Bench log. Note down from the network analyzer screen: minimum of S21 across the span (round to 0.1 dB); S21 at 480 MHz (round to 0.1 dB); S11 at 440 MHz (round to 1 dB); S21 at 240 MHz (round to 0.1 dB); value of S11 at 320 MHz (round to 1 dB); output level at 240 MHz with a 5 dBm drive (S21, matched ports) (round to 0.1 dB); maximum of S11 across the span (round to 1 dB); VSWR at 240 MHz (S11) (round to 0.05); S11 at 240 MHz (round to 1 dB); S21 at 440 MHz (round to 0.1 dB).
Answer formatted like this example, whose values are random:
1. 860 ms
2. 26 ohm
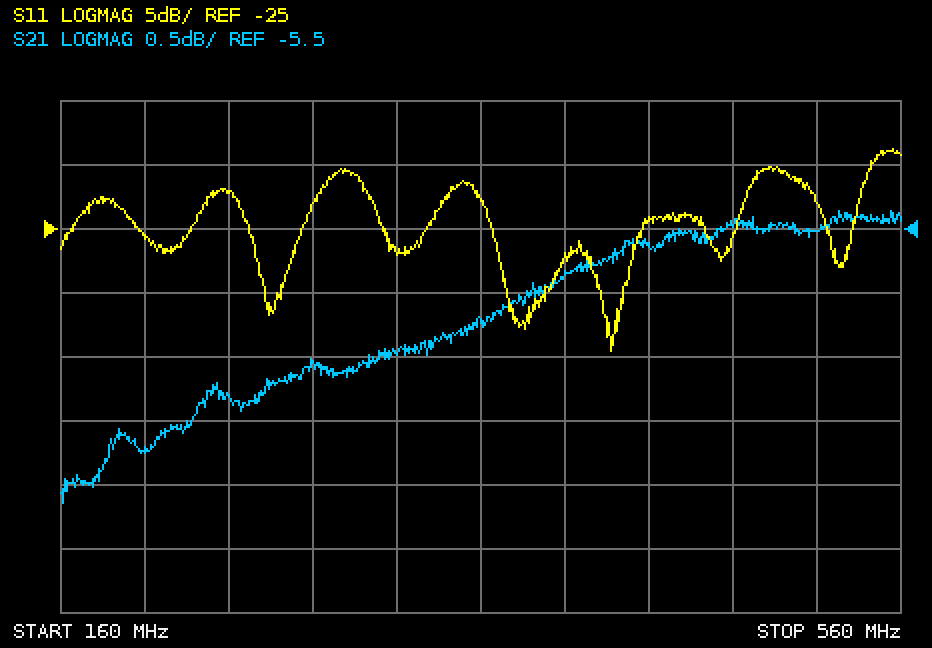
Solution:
1. -7.6 dB
2. -5.5 dB
3. -24 dB
4. -6.8 dB
5. -27 dB
6. -1.8 dBm
7. -19 dB
8. 1.15
9. -22 dB
10. -5.6 dB
